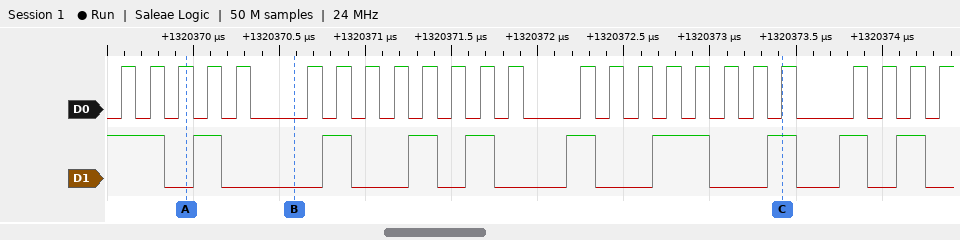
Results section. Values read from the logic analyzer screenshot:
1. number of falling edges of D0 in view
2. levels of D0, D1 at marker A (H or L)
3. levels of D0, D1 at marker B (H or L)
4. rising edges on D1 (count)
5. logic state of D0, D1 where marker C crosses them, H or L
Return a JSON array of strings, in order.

["24", "D0=H, D1=L", "D0=L, D1=L", "9", "D0=H, D1=H"]
